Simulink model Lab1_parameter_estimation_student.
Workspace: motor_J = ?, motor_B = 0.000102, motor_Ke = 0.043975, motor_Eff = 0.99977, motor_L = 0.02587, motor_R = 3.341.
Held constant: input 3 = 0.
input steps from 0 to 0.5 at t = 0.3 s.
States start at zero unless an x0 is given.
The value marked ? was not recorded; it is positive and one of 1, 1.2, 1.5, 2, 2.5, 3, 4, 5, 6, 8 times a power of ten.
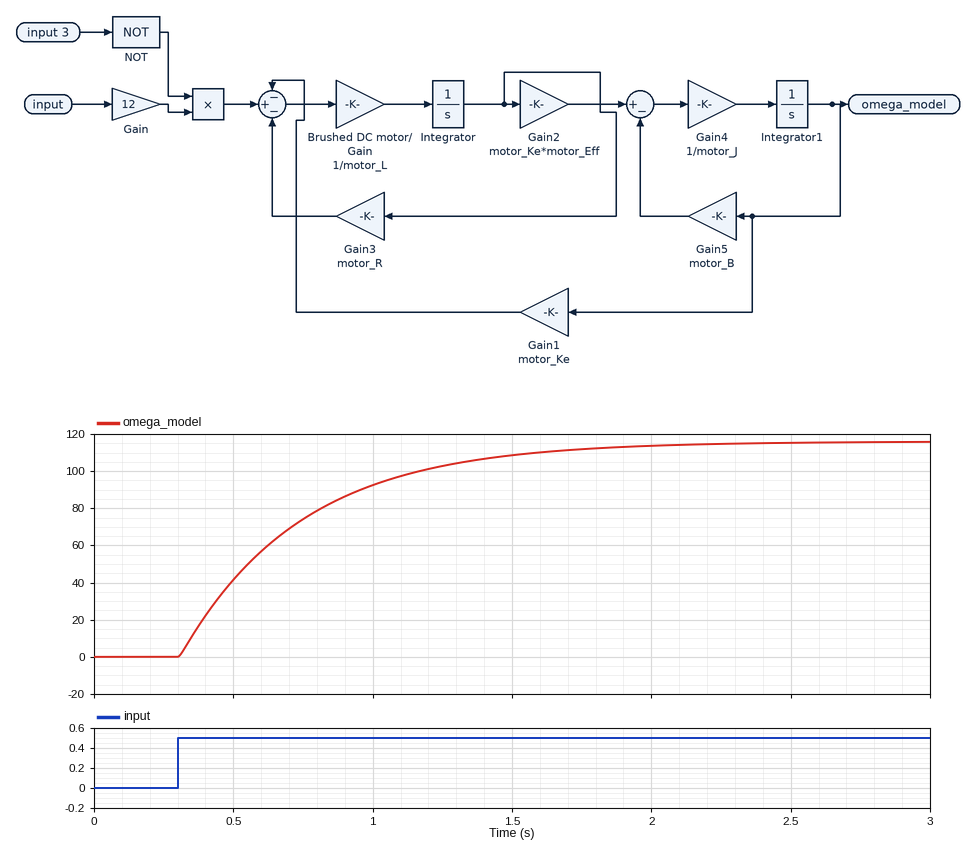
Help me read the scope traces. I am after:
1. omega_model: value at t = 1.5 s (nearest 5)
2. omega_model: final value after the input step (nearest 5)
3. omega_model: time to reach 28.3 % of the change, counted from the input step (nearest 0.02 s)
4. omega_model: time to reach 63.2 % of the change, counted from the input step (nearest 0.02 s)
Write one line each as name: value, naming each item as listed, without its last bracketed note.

omega_model: value at t = 1.5 s: 110
omega_model: final value after the input step: 115
omega_model: time to reach 28.3 % of the change, counted from the input step: 0.16 s
omega_model: time to reach 63.2 % of the change, counted from the input step: 0.44 s
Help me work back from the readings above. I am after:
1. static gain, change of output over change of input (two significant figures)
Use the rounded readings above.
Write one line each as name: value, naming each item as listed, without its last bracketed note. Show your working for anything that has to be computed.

static gain, change of output over change of input: (115 - 0) / (0.5 - 0) = 230
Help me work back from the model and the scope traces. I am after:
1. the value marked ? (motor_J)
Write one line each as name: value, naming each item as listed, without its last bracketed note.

the value marked ?: 0.0003
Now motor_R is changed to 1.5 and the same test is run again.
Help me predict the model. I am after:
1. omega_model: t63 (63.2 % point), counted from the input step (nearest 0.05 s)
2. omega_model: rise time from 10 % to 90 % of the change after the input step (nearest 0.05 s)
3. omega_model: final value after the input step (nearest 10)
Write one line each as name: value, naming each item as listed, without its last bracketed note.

omega_model: t63 (63.2 % point), counted from the input step: 0.20 s
omega_model: rise time from 10 % to 90 % of the change after the input step: 0.45 s
omega_model: final value after the input step: 130
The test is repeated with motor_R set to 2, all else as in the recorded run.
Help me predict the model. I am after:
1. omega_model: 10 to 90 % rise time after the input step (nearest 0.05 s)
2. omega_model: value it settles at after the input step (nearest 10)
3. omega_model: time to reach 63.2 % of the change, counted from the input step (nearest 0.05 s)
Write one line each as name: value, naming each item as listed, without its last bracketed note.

omega_model: 10 to 90 % rise time after the input step: 0.60 s
omega_model: value it settles at after the input step: 120
omega_model: time to reach 63.2 % of the change, counted from the input step: 0.30 s
